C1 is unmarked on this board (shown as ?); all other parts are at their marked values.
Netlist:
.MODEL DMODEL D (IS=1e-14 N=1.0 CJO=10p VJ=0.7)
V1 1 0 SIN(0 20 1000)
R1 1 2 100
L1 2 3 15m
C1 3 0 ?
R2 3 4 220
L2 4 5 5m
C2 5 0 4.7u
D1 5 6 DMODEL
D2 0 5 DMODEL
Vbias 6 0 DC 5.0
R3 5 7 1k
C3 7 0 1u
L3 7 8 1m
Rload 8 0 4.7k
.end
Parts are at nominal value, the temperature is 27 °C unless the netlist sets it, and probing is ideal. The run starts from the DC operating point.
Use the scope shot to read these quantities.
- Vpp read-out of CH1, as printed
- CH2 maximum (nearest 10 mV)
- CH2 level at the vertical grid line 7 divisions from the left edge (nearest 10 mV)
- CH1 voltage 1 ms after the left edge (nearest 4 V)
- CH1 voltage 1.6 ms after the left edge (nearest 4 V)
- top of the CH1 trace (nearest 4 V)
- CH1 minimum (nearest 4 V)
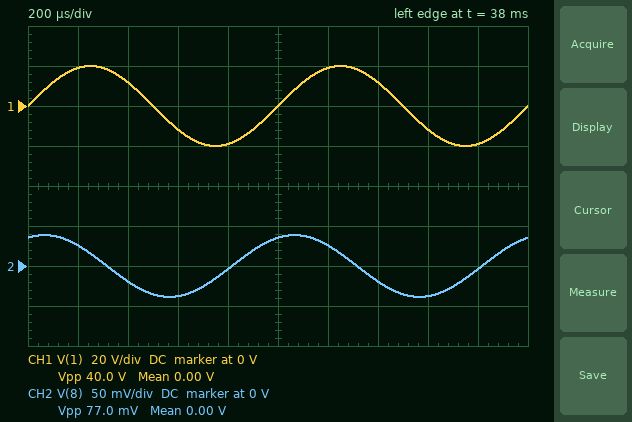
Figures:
40.0 V
40 mV
-20 mV
0 V
-12 V
20 V
-20 V
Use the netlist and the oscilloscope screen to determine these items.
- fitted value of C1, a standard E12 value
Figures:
15 µF
